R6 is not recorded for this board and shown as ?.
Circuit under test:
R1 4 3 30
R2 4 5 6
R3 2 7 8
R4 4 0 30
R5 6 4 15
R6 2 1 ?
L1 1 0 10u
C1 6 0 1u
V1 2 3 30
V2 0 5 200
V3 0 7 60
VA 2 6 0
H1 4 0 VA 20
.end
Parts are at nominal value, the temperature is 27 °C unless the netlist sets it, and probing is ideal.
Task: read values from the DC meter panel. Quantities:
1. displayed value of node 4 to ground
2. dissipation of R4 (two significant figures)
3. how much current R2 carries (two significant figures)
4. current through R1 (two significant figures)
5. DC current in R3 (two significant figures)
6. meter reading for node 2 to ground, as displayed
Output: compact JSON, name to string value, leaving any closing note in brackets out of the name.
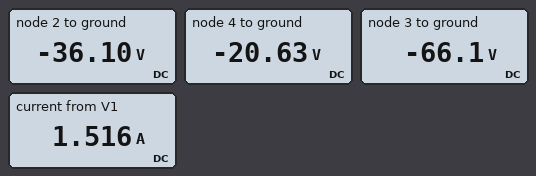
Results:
{"displayed value of node 4 to ground": "-20.63 V", "dissipation of R4": "14 W", "how much current R2 carries": "30 A", "current through R1": "1.5 A", "DC current in R3": "3.0 A", "meter reading for node 2 to ground, as displayed": "-36.10 V"}
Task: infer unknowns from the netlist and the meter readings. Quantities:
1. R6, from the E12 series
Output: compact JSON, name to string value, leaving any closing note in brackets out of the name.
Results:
{"R6, from the E12 series": "82 Ω"}
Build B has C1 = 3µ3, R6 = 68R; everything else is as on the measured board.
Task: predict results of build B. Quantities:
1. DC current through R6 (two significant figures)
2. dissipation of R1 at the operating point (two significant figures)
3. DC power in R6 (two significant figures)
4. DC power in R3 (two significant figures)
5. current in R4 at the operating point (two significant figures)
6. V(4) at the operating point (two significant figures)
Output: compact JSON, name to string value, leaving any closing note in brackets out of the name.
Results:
{"DC current through R6": "520 mA", "dissipation of R1 at the operating point": "68 W", "DC power in R6": "19 W", "DC power in R3": "74 W", "current in R4 at the operating point": "680 mA", "V(4) at the operating point": "-20 V"}
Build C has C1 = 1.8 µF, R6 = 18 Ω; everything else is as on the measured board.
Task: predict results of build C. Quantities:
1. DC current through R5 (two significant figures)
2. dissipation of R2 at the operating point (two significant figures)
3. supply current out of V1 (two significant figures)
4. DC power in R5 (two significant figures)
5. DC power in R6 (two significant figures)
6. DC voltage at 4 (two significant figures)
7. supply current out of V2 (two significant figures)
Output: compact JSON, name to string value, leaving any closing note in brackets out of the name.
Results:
{"DC current through R5": "830 mA", "dissipation of R2 at the operating point": "5.6 kW", "supply current out of V1": "1.4 A", "DC power in R5": "10 W", "DC power in R6": "47 W", "DC voltage at 4": "-17 V", "supply current out of V2": "31 A"}
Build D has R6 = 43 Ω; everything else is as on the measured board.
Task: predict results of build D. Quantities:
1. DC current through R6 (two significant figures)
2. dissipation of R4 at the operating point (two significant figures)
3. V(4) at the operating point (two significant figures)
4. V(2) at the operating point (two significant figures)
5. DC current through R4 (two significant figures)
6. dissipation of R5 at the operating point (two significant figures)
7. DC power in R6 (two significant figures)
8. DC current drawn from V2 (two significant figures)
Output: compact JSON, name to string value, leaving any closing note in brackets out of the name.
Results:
{"DC current through R6": "790 mA", "dissipation of R4 at the operating point": "13 W", "V(4) at the operating point": "-19 V", "V(2) at the operating point": "-34 V", "DC current through R4": "650 mA", "dissipation of R5 at the operating point": "14 W", "DC power in R6": "27 W", "DC current drawn from V2": "30 A"}
